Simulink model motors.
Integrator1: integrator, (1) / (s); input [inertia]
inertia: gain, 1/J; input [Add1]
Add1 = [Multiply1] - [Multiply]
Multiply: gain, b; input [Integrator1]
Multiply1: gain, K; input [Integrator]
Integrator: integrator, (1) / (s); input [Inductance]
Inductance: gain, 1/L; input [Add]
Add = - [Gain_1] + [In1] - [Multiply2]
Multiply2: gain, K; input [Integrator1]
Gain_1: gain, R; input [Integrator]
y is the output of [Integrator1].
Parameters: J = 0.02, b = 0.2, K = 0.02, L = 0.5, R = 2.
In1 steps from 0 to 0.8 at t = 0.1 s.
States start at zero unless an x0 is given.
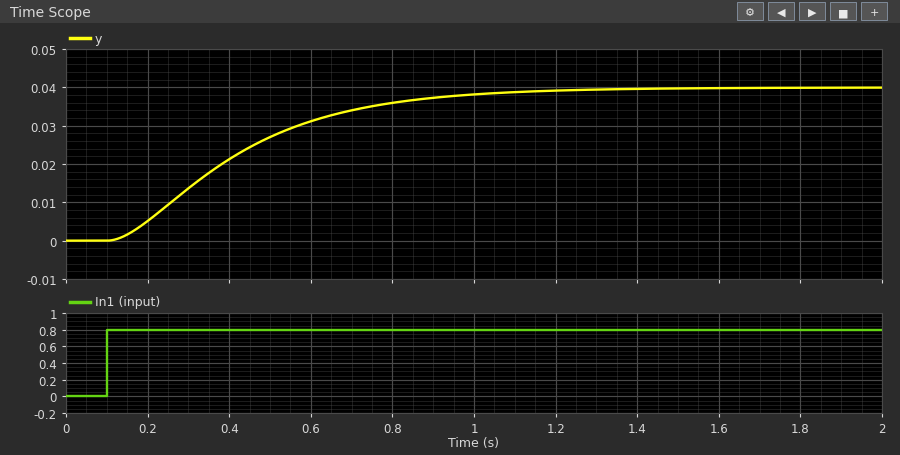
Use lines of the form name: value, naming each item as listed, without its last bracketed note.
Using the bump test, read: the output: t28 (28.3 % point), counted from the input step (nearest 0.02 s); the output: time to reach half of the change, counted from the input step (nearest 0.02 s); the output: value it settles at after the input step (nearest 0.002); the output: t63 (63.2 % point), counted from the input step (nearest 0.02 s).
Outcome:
the output: t28 (28.3 % point), counted from the input step: 0.18 s
the output: time to reach half of the change, counted from the input step: 0.28 s
the output: value it settles at after the input step: 0.040
the output: t63 (63.2 % point), counted from the input step: 0.36 s
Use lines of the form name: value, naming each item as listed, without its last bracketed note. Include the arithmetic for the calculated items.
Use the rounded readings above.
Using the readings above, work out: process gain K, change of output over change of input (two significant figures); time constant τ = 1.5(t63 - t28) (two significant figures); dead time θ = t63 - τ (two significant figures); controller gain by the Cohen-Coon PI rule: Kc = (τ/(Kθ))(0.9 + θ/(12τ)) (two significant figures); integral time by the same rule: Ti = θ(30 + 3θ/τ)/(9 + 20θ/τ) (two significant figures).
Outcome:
process gain K, change of output over change of input: (0.04 - 0) / 0.8 = 0.050
time constant τ = 1.5(t63 - t28): 1.5 × (0.36 - 0.18) = 0.27 s
dead time θ = t63 - τ: 0.36 - 0.27 = 0.090 s
controller gain by the Cohen-Coon PI rule: Kc = (τ/(Kθ))(0.9 + θ/(12τ)): 0.27 / (0.05 × 0.09) × (0.9 + 0.09 / (12 × 0.27)) = 56
integral time by the same rule: Ti = θ(30 + 3θ/τ)/(9 + 20θ/τ): 0.09 × (30 + 3 × 0.09 / 0.27) / (9 + 20 × 0.09 / 0.27) = 0.18 s
